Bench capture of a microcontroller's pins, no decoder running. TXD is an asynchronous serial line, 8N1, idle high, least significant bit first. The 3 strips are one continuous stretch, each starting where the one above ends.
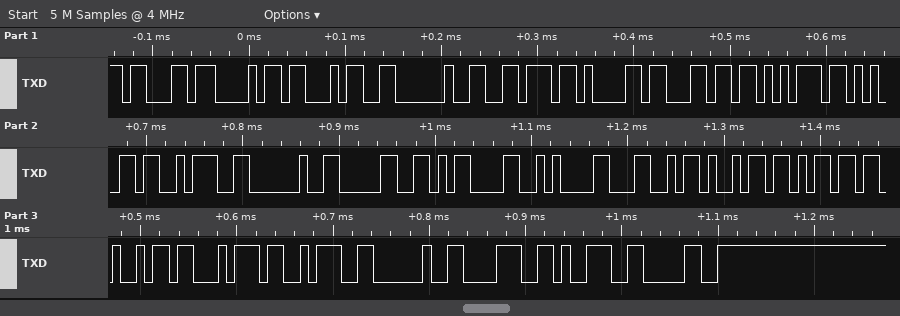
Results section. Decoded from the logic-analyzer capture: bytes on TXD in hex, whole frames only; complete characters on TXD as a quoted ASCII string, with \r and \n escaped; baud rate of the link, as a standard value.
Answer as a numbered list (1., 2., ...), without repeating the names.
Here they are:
1. 0x63 0x68 0x34 0x20 0x76 0x61 0x6C 0x75 0x65 0x3A 0x20 0x30 0x0D 0x0A 0x4C 0x69 0x6D 0x69 0x74 0x3A 0x20 0x38 0x39 0x30
2. "ch4 value: 0\r\nLimit: 890"
3. 115200 baud
